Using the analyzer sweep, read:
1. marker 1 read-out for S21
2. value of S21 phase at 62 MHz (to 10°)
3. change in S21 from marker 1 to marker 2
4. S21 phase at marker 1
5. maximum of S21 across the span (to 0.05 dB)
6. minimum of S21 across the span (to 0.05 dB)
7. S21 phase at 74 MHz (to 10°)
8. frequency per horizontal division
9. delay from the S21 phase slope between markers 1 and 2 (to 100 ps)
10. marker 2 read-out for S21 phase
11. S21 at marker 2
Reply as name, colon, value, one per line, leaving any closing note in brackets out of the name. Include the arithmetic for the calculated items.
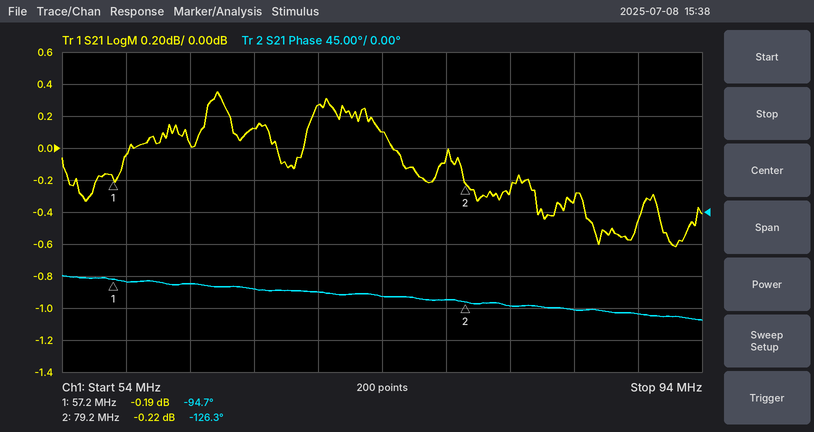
marker 1 read-out for S21: -0.19 dB
value of S21 phase at 62 MHz: -100°
change in S21 from marker 1 to marker 2: -0.22 − (-0.19) = -0.03 dB
S21 phase at marker 1: -94.7°
maximum of S21 across the span: 0.35 dB
minimum of S21 across the span: -0.60 dB
S21 phase at 74 MHz: -120°
frequency per horizontal division: 4 MHz
delay from the S21 phase slope between markers 1 and 2: −(-126.3° − (-94.7°))/(360° × 22 MHz) ≈ 4.0 ns
marker 2 read-out for S21 phase: -126.3°
S21 at marker 2: -0.22 dB
